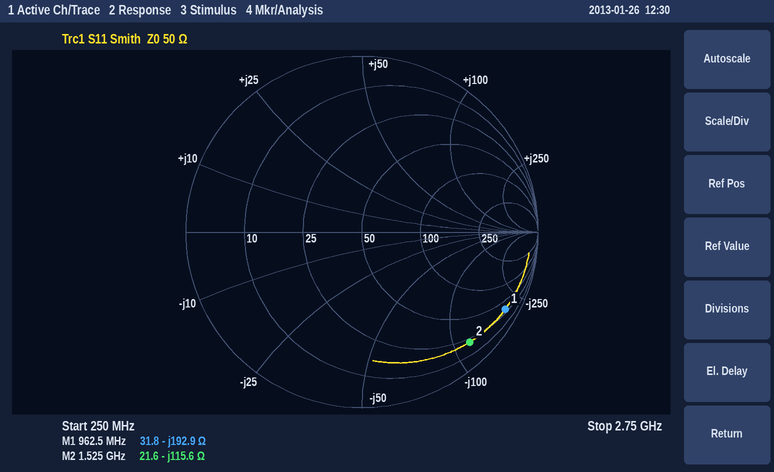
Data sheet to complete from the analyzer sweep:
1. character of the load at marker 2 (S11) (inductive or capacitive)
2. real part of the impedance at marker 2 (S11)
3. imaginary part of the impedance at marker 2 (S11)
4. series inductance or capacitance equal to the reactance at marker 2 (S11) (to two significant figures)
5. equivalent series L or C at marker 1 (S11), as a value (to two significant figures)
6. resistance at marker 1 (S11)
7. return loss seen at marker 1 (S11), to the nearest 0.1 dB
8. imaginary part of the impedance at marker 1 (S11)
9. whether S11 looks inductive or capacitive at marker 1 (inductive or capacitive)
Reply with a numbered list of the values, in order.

1. capacitive
2. 21.6 Ω
3. -115.6 Ω
4. 900 fF
5. 860 fF
6. 31.8 Ω
7. 0.7 dB
8. -192.9 Ω
9. capacitive
